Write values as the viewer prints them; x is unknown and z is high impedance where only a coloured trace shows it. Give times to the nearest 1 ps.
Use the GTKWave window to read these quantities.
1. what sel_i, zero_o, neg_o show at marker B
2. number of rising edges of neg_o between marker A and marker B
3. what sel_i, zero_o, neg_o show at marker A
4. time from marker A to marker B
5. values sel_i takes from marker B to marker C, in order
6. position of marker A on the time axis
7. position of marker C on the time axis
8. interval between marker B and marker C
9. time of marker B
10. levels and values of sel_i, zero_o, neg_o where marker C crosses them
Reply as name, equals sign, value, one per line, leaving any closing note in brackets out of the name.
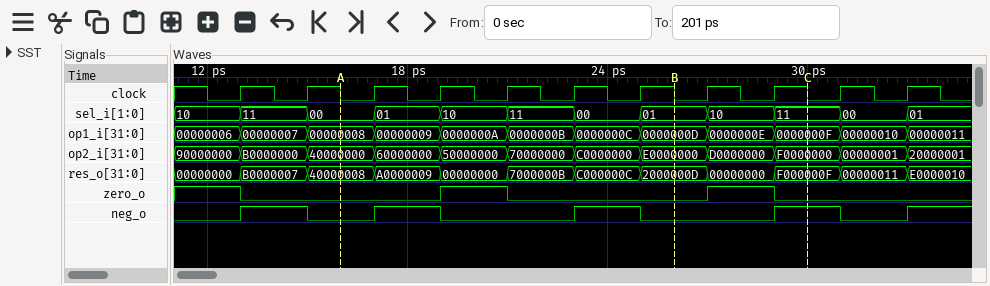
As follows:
what sel_i, zero_o, neg_o show at marker B = sel_i=01, zero_o=0, neg_o=0
number of rising edges of neg_o between marker A and marker B = 2
what sel_i, zero_o, neg_o show at marker A = sel_i=00, zero_o=0, neg_o=0
time from marker A to marker B = 10 ps
values sel_i takes from marker B to marker C, in order = 01, 10, 11
position of marker A on the time axis = 16 ps
position of marker C on the time axis = 30 ps
interval between marker B and marker C = 4 ps
time of marker B = 26 ps
levels and values of sel_i, zero_o, neg_o where marker C crosses them = sel_i=11, zero_o=0, neg_o=1
